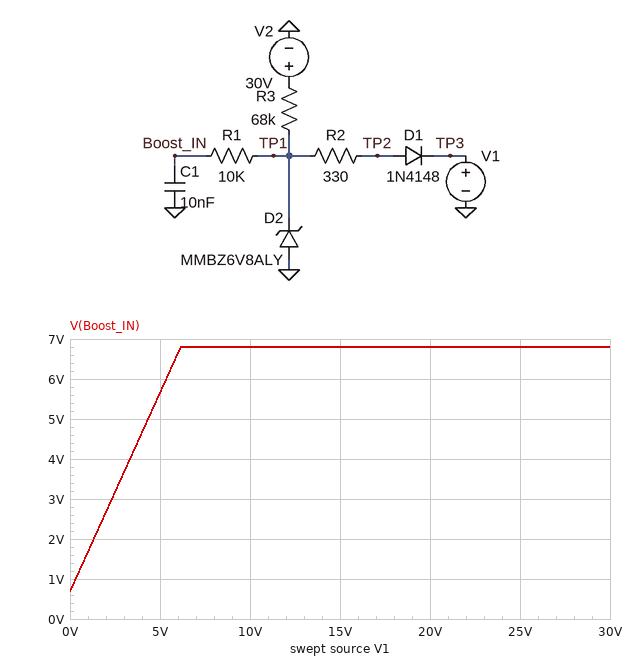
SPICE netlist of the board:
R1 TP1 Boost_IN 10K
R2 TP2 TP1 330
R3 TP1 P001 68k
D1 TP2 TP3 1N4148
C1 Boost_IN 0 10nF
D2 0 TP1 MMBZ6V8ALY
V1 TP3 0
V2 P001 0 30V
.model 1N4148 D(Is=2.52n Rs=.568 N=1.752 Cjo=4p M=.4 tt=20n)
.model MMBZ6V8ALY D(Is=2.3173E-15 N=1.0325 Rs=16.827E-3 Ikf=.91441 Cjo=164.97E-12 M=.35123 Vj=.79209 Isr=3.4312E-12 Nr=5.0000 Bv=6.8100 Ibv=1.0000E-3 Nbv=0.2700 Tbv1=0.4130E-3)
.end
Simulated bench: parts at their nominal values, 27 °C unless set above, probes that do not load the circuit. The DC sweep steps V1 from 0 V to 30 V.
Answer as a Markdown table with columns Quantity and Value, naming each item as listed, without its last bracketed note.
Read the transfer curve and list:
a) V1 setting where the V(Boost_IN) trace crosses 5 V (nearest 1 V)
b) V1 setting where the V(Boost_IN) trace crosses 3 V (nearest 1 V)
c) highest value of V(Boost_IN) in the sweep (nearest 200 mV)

| Quantity | Value |
|---|---|
| V1 setting where the V(Boost_IN) trace crosses 5 V | 4 V |
| V1 setting where the V(Boost_IN) trace crosses 3 V | 2 V |
| highest value of V(Boost_IN) in the sweep | 6.8 V |
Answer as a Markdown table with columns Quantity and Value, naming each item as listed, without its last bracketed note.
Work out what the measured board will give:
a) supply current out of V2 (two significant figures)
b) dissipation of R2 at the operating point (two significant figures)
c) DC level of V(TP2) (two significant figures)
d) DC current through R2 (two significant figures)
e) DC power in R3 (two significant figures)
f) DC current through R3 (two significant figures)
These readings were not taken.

| Quantity | Value |
|---|---|
| supply current out of V2 | 430 µA |
| dissipation of R2 at the operating point | 61 µW |
| DC level of V(TP2) | 550 mV |
| DC current through R2 | 430 µA |
| DC power in R3 | 13 mW |
| DC current through R3 | 430 µA |
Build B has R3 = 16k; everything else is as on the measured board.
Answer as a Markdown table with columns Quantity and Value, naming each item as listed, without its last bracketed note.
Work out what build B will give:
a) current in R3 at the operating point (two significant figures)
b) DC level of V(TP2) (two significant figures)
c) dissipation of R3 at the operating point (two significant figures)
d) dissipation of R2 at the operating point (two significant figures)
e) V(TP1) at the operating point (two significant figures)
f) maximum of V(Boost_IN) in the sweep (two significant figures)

| Quantity | Value |
|---|---|
| current in R3 at the operating point | 1.8 mA |
| DC level of V(TP2) | 610 mV |
| dissipation of R3 at the operating point | 52 mW |
| dissipation of R2 at the operating point | 1.1 mW |
| V(TP1) at the operating point | 1.2 V |
| maximum of V(Boost_IN) in the sweep | 6.8 V |
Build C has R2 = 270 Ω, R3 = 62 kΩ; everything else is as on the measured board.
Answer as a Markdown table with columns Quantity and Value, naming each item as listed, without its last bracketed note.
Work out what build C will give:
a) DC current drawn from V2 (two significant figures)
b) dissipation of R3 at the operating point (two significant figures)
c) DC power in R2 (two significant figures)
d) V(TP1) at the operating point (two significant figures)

| Quantity | Value |
|---|---|
| DC current drawn from V2 | 470 µA |
| dissipation of R3 at the operating point | 14 mW |
| DC power in R2 | 60 µW |
| V(TP1) at the operating point | 680 mV |
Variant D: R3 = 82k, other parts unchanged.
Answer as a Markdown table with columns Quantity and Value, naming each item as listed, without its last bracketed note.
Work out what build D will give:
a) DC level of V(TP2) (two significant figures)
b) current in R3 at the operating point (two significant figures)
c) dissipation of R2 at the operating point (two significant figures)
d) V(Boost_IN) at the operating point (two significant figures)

| Quantity | Value |
|---|---|
| DC level of V(TP2) | 540 mV |
| current in R3 at the operating point | 360 µA |
| dissipation of R2 at the operating point | 42 µW |
| V(Boost_IN) at the operating point | 660 mV |
